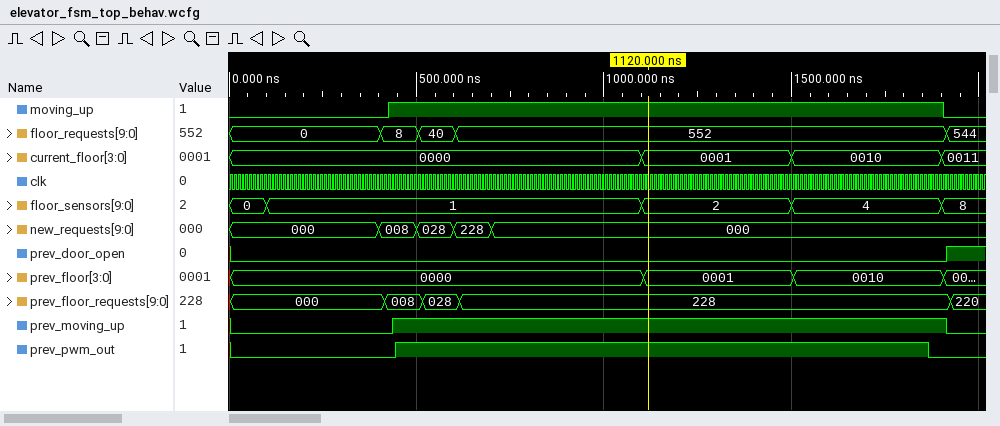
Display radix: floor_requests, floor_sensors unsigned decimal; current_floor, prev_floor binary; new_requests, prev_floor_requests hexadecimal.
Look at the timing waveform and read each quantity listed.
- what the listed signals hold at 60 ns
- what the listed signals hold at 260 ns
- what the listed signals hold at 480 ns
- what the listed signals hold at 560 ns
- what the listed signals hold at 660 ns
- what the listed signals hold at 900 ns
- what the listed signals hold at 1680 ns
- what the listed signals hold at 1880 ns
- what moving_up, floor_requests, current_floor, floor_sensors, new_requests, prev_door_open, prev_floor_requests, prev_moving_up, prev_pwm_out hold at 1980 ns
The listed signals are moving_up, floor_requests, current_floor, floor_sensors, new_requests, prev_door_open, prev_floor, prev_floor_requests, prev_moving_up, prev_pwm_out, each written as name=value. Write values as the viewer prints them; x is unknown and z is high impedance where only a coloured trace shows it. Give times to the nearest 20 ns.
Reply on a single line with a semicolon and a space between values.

moving_up=0, floor_requests=0, current_floor=0000, floor_sensors=0, new_requests=000, prev_door_open=0, prev_floor=0000, prev_floor_requests=000, prev_moving_up=0, prev_pwm_out=0; moving_up=0, floor_requests=0, current_floor=0000, floor_sensors=1, new_requests=000, prev_door_open=0, prev_floor=0000, prev_floor_requests=000, prev_moving_up=0, prev_pwm_out=0; moving_up=1, floor_requests=8, current_floor=0000, floor_sensors=1, new_requests=008, prev_door_open=0, prev_floor=0000, prev_floor_requests=008, prev_moving_up=1, prev_pwm_out=1; moving_up=1, floor_requests=40, current_floor=0000, floor_sensors=1, new_requests=028, prev_door_open=0, prev_floor=0000, prev_floor_requests=028, prev_moving_up=1, prev_pwm_out=1; moving_up=1, floor_requests=552, current_floor=0000, floor_sensors=1, new_requests=228, prev_door_open=0, prev_floor=0000, prev_floor_requests=228, prev_moving_up=1, prev_pwm_out=1; moving_up=1, floor_requests=552, current_floor=0000, floor_sensors=1, new_requests=000, prev_door_open=0, prev_floor=0000, prev_floor_requests=228, prev_moving_up=1, prev_pwm_out=1; moving_up=1, floor_requests=552, current_floor=0010, floor_sensors=4, new_requests=000, prev_door_open=0, prev_floor=0010, prev_floor_requests=228, prev_moving_up=1, prev_pwm_out=1; moving_up=1, floor_requests=552, current_floor=0010, floor_sensors=4, new_requests=000, prev_door_open=0, prev_floor=0010, prev_floor_requests=228, prev_moving_up=1, prev_pwm_out=0; moving_up=0, floor_requests=544, current_floor=0011, floor_sensors=8, new_requests=000, prev_door_open=1, prev_floor_requests=220, prev_moving_up=0, prev_pwm_out=0
